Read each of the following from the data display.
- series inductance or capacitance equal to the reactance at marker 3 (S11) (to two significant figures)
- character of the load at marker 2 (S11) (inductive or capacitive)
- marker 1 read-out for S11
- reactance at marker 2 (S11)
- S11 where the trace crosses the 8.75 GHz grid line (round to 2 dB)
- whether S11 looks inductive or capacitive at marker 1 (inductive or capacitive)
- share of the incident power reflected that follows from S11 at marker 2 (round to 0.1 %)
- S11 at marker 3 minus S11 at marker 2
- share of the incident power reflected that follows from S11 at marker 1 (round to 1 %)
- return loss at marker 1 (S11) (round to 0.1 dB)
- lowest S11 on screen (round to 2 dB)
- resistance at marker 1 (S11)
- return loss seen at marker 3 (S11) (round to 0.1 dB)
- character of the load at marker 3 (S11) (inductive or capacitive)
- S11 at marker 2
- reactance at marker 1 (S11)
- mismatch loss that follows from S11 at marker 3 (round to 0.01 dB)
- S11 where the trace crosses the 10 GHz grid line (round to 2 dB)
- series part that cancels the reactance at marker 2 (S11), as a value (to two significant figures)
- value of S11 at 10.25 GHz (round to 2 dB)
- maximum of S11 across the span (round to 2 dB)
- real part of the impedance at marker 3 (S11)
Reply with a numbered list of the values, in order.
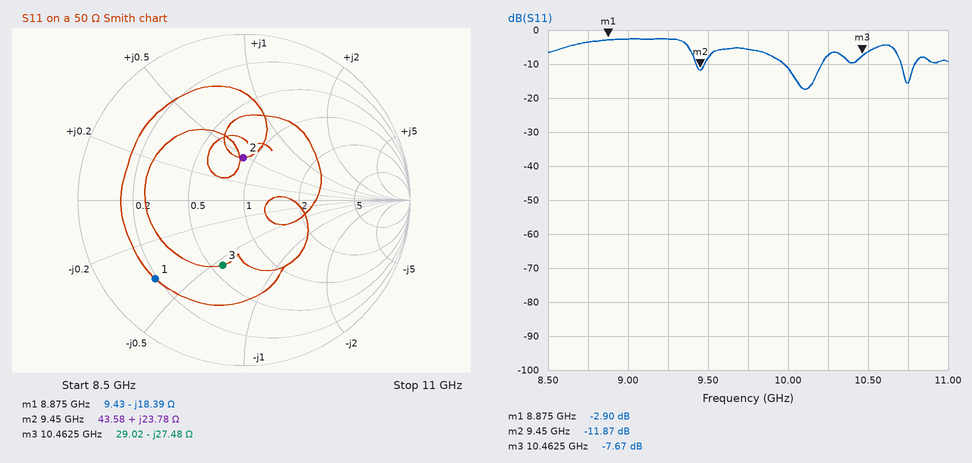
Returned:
1. 550 fF
2. inductive
3. -2.90 dB
4. +23.78 Ω
5. -4 dB
6. capacitive
7. 6.5 %
8. 4.20 dB
9. 51 %
10. 2.9 dB
11. -18 dB
12. 9.43 Ω
13. 7.7 dB
14. capacitive
15. -11.87 dB
16. -18.39 Ω
17. 0.81 dB
18. -12 dB
19. 710 fF
20. -8 dB
21. -2 dB
22. 29.02 Ω
